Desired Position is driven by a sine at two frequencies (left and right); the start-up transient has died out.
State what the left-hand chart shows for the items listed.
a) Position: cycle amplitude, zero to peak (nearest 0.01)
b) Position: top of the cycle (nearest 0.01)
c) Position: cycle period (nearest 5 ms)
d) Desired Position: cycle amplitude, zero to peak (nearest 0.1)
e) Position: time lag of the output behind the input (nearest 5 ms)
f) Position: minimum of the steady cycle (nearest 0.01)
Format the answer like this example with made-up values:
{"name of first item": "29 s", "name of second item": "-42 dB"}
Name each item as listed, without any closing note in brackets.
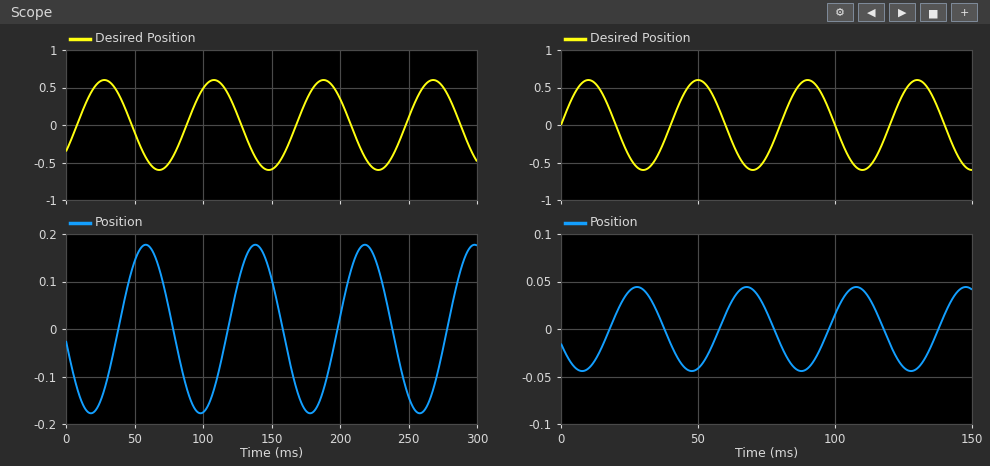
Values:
{"Position: cycle amplitude, zero to peak": "0.18", "Position: top of the cycle": "0.18", "Position: cycle period": "80 ms", "Desired Position: cycle amplitude, zero to peak": "0.6", "Position: time lag of the output behind the input": "30 ms", "Position: minimum of the steady cycle": "-0.18"}
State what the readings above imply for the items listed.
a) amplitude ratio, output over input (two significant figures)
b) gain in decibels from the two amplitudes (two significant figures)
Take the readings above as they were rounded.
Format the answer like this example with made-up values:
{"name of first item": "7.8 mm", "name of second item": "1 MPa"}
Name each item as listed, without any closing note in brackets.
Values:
{"amplitude ratio, output over input": "0.30", "gain in decibels from the two amplitudes": "-10 dB"}
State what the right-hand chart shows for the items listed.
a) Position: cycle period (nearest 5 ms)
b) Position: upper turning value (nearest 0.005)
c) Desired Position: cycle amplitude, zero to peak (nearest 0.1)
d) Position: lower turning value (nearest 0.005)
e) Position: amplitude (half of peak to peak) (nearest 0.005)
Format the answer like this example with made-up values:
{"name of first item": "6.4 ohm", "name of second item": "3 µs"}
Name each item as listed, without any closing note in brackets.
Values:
{"Position: cycle period": "40 ms", "Position: upper turning value": "0.045", "Desired Position: cycle amplitude, zero to peak": "0.6", "Position: lower turning value": "-0.045", "Position: amplitude (half of peak to peak)": "0.045"}
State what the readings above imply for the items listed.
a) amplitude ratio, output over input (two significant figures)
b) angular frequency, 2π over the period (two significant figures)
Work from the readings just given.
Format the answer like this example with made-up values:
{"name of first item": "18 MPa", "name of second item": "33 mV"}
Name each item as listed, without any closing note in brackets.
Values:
{"amplitude ratio, output over input": "0.075", "angular frequency, 2π over the period": "0.16 rad/ms"}
